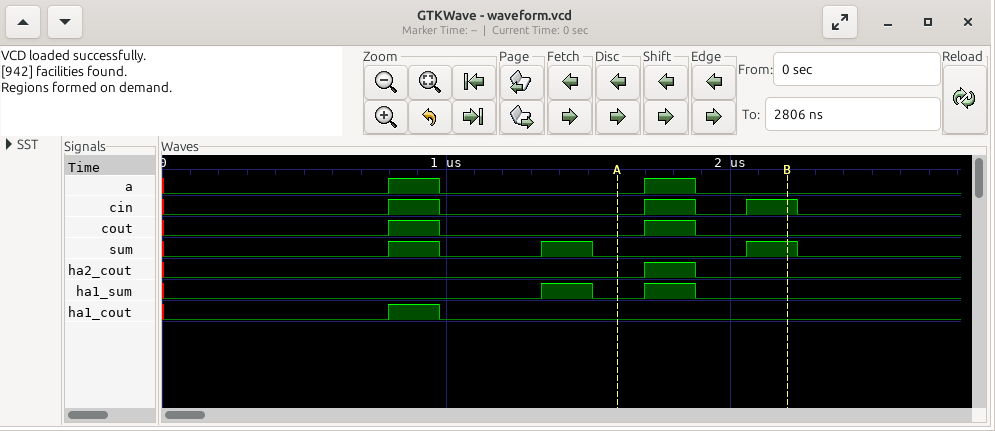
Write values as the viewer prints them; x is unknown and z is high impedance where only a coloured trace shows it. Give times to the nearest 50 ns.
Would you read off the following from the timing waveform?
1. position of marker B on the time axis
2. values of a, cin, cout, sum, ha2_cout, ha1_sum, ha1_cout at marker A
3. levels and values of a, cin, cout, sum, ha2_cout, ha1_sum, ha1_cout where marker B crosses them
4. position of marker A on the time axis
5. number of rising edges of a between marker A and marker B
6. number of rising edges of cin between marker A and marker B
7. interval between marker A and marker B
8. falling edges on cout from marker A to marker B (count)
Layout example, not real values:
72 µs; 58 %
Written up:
2200 ns; a=0, cin=0, cout=0, sum=0, ha2_cout=0, ha1_sum=0, ha1_cout=0; a=0, cin=1, cout=0, sum=1, ha2_cout=0, ha1_sum=0, ha1_cout=0; 1600 ns; 1; 2; 600 ns; 1
